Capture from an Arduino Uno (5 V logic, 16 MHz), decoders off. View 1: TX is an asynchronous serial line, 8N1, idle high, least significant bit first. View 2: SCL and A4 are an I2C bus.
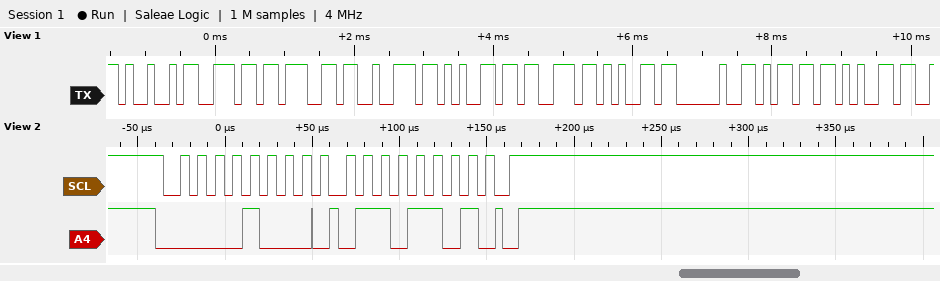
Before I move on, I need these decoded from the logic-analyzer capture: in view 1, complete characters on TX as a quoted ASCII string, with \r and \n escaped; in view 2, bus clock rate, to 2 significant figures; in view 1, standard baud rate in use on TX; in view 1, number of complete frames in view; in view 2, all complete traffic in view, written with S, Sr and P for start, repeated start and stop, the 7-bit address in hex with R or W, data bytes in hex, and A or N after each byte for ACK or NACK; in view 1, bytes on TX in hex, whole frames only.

"Ingrese me"
100 kHz
9600 baud
10
S 04W A 6D A P
49 6E 67 72 65 73 65 20 6D 65
